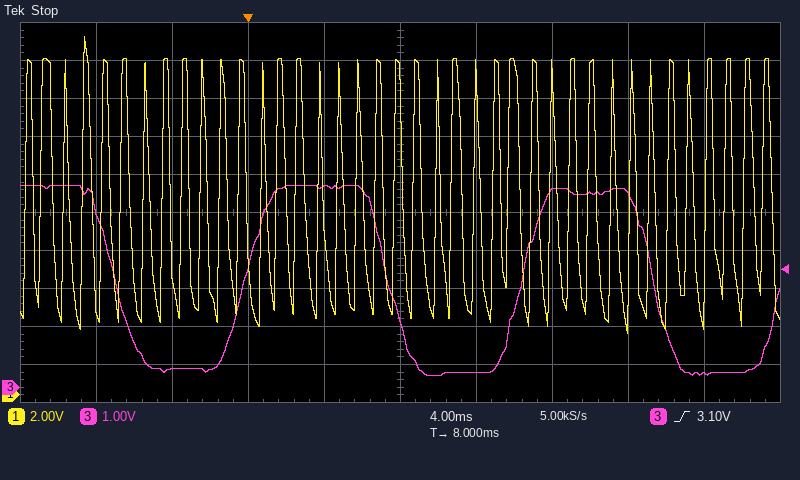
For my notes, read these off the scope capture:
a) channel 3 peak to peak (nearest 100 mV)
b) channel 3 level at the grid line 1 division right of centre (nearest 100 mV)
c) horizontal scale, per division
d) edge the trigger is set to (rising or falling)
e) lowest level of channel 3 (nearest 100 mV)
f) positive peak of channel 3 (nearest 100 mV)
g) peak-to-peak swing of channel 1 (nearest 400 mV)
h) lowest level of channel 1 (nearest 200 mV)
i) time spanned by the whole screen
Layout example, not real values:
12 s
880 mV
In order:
5.0 V
400 mV
4 ms
rising
300 mV
5.3 V
15.6 V
3.2 V
40 ms
